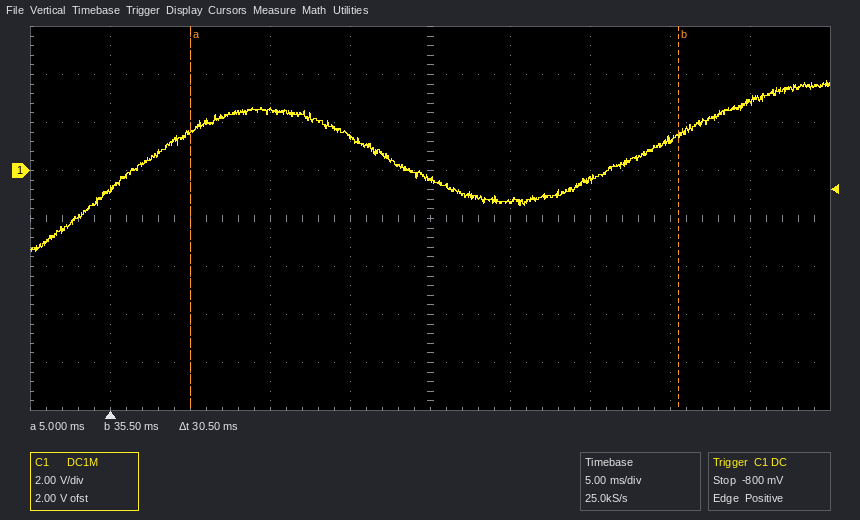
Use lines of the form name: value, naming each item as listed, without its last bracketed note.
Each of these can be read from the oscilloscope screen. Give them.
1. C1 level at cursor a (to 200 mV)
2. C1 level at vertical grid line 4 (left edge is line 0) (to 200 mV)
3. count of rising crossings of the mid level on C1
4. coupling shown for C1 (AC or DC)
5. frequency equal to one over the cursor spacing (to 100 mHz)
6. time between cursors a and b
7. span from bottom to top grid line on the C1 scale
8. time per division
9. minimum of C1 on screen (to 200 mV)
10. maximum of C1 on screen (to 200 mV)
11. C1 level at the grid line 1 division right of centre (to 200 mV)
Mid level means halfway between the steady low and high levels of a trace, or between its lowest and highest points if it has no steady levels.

C1 level at cursor a: 1.6 V
C1 level at vertical grid line 4 (left edge is line 0): 1.4 V
count of rising crossings of the mid level on C1: 2
coupling shown for C1: DC
frequency equal to one over the cursor spacing: 32.8 Hz
time between cursors a and b: 30.5 ms
span from bottom to top grid line on the C1 scale: 16 V
time per division: 5 ms
minimum of C1 on screen: -3.4 V
maximum of C1 on screen: 3.8 V
C1 level at the grid line 1 division right of centre: -1.2 V
